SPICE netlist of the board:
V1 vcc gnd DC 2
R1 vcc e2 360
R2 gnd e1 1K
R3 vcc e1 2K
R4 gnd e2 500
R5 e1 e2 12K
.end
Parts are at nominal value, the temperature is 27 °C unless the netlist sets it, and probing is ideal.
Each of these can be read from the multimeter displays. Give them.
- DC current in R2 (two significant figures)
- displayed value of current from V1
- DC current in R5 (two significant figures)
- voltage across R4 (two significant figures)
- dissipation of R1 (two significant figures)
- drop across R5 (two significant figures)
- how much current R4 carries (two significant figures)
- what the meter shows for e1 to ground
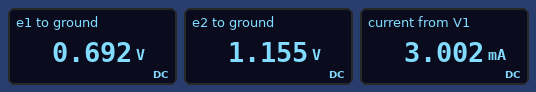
690 µA
3.002 mA
39 µA
1.2 V
2.0 mW
460 mV
2.3 mA
0.692 V
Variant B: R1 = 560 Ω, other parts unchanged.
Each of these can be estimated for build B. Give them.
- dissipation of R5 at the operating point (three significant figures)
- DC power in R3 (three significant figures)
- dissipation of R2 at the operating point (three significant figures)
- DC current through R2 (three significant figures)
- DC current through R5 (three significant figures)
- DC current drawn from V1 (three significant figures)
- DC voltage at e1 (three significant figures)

5.50 µW
870 µW
464 µW
681 µA
21.4 µA
2.56 mA
681 mV
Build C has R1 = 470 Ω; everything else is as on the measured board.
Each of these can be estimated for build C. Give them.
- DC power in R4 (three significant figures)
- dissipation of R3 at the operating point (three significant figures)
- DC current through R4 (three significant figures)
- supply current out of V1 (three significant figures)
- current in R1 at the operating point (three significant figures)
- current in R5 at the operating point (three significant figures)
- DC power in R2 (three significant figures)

2.10 mW
864 µW
2.05 mA
2.73 mA
2.08 mA
28.2 µA
470 µW
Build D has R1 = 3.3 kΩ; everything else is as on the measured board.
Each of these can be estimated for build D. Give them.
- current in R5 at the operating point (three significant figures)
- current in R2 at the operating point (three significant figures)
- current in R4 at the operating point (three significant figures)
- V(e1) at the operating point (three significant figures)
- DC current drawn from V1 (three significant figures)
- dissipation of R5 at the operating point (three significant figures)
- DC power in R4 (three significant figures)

30.8 µA
646 µA
553 µA
646 mV
1.20 mA
11.4 µW
153 µW
